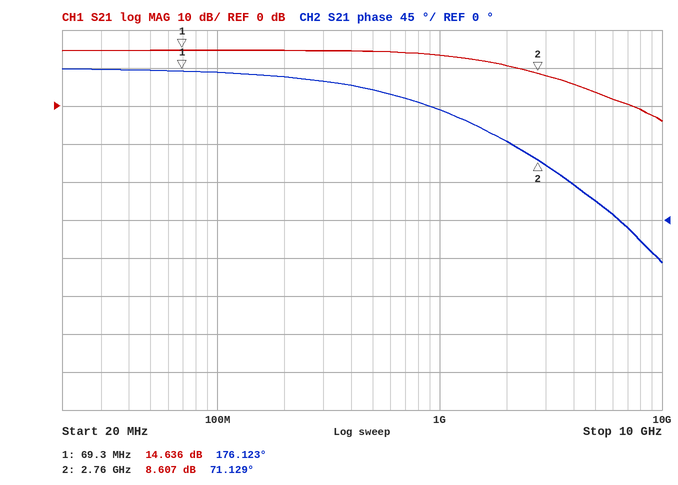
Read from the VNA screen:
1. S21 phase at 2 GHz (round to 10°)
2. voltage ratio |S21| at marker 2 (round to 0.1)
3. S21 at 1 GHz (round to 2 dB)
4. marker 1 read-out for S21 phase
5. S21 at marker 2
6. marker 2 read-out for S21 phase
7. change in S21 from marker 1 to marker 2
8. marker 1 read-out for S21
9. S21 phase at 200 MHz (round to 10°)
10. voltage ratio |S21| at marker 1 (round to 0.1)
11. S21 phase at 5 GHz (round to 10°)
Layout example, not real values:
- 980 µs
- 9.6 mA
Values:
- 90°
- 2.7
- 14 dB
- 176.123°
- 8.607 dB
- 71.129°
- -6.029 dB
- 14.636 dB
- 170°
- 5.4
- 20°
